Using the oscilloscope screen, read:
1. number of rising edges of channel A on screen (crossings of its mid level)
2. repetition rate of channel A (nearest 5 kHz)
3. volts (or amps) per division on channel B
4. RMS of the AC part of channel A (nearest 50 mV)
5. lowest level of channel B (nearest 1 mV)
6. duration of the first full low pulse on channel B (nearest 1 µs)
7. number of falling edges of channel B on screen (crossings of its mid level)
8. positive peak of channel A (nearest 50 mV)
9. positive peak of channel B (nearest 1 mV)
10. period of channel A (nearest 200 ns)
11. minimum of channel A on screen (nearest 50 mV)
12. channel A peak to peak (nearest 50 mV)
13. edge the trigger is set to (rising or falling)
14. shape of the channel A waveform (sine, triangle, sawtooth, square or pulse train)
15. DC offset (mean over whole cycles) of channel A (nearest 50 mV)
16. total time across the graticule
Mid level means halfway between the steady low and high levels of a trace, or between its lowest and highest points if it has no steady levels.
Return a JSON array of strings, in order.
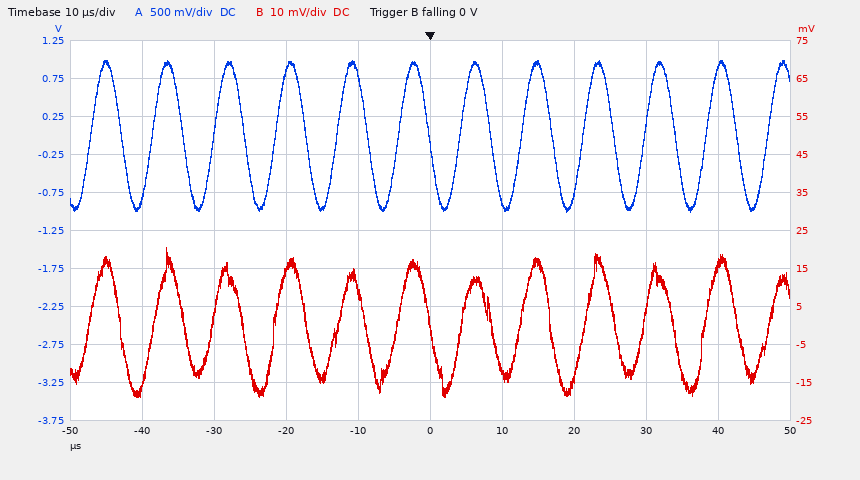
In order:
["12", "115 kHz", "10 mV", "700 mV", "-19 mV", "5 µs", "11", "1.00 V", "21 mV", "8.6 µs", "-1.00 V", "2.00 V", "falling", "sine", "0 mV", "100 µs"]
